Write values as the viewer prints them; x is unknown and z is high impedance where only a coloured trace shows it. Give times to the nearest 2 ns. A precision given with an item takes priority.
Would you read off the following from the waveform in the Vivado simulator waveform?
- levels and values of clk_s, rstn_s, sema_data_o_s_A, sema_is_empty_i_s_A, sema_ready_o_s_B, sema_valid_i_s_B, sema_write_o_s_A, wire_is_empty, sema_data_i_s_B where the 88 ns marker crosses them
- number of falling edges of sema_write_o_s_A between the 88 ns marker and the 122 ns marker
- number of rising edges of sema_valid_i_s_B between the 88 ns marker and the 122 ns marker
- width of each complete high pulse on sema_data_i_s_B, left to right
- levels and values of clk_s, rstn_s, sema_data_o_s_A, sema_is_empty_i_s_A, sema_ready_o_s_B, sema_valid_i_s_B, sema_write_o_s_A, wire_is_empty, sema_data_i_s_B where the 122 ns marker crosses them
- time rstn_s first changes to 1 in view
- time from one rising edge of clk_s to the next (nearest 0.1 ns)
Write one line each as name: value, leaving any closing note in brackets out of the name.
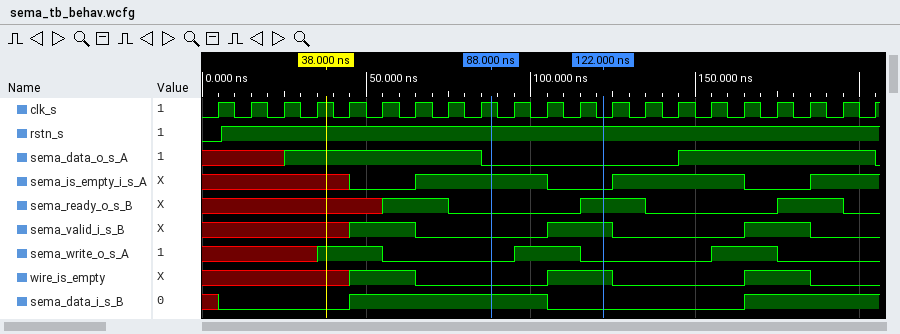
levels and values of clk_s, rstn_s, sema_data_o_s_A, sema_is_empty_i_s_A, sema_ready_o_s_B, sema_valid_i_s_B, sema_write_o_s_A, wire_is_empty, sema_data_i_s_B where the 88 ns marker crosses them: clk_s=1, rstn_s=1, sema_data_o_s_A=0, sema_is_empty_i_s_A=1, sema_ready_o_s_B=0, sema_valid_i_s_B=0, sema_write_o_s_A=0, wire_is_empty=0, sema_data_i_s_B=1
number of falling edges of sema_write_o_s_A between the 88 ns marker and the 122 ns marker: 1
number of rising edges of sema_valid_i_s_B between the 88 ns marker and the 122 ns marker: 1
width of each complete high pulse on sema_data_i_s_B, left to right: 60 ns
levels and values of clk_s, rstn_s, sema_data_o_s_A, sema_is_empty_i_s_A, sema_ready_o_s_B, sema_valid_i_s_B, sema_write_o_s_A, wire_is_empty, sema_data_i_s_B where the 122 ns marker crosses them: clk_s=0, rstn_s=1, sema_data_o_s_A=0, sema_is_empty_i_s_A=0, sema_ready_o_s_B=1, sema_valid_i_s_B=1, sema_write_o_s_A=0, wire_is_empty=1, sema_data_i_s_B=0
time rstn_s first changes to 1 in view: 6 ns
time from one rising edge of clk_s to the next: 10 ns
